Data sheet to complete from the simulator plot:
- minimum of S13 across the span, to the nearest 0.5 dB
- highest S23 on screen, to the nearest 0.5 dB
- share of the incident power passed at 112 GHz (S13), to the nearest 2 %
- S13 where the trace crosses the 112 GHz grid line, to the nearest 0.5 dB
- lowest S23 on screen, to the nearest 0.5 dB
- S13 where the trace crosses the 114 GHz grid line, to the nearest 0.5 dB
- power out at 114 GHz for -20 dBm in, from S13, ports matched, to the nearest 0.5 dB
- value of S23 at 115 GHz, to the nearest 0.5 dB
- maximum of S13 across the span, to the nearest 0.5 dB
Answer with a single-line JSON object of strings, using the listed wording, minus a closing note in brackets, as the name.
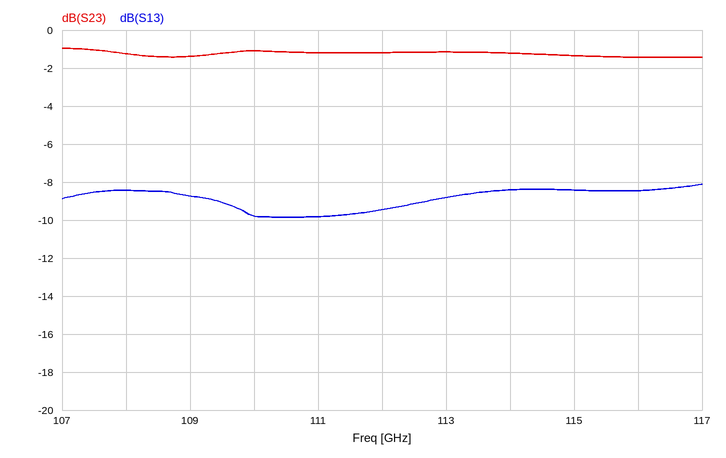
{"minimum of S13 across the span, to the nearest 0.5 dB": "-10.0 dB", "highest S23 on screen, to the nearest 0.5 dB": "-1.0 dB", "share of the incident power passed at 112 GHz (S13), to the nearest 2 %": "12 %", "S13 where the trace crosses the 112 GHz grid line, to the nearest 0.5 dB": "-9.5 dB", "lowest S23 on screen, to the nearest 0.5 dB": "-1.5 dB", "S13 where the trace crosses the 114 GHz grid line, to the nearest 0.5 dB": "-8.5 dB", "power out at 114 GHz for -20 dBm in, from S13, ports matched, to the nearest 0.5 dB": "-28.5 dBm", "value of S23 at 115 GHz, to the nearest 0.5 dB": "-1.5 dB", "maximum of S13 across the span, to the nearest 0.5 dB": "-8.0 dB"}
